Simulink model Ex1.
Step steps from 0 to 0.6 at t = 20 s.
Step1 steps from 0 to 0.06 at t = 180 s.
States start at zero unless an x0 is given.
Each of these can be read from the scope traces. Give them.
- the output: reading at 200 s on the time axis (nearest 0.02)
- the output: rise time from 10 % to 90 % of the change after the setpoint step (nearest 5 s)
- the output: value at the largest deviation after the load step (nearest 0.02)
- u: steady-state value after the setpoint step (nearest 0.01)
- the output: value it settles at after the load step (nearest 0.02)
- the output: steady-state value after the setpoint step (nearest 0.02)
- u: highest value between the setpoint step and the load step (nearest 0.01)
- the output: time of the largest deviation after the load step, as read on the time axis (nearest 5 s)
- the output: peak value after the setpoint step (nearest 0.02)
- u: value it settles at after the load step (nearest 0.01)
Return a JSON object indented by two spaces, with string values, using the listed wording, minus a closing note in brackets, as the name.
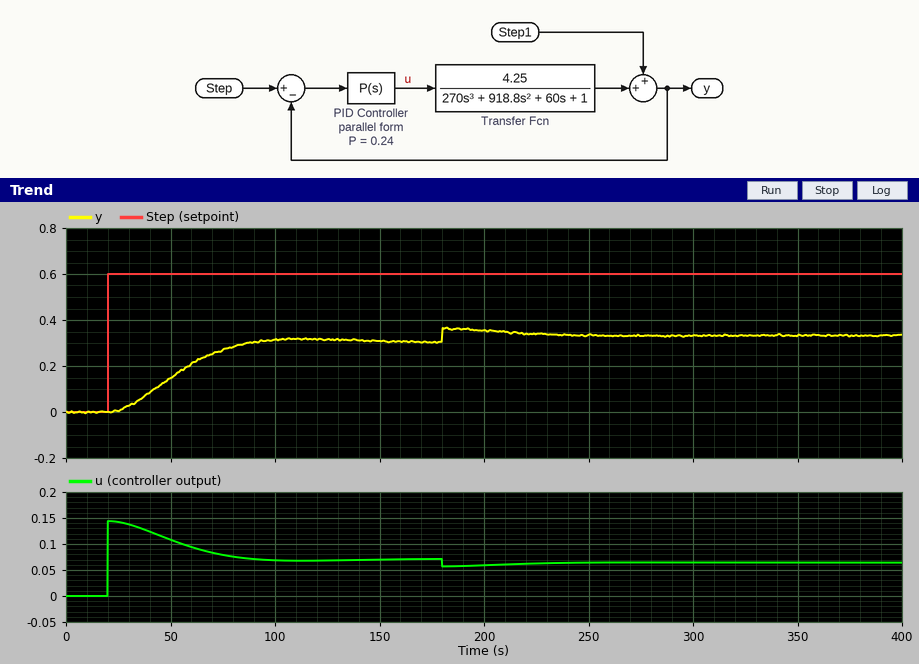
{
  "the output: reading at 200 s on the time axis": "0.36",
  "the output: rise time from 10 % to 90 % of the change after the setpoint step": "45 s",
  "the output: value at the largest deviation after the load step": "0.36",
  "u: steady-state value after the setpoint step": "0.07",
  "the output: value it settles at after the load step": "0.34",
  "the output: steady-state value after the setpoint step": "0.30",
  "u: highest value between the setpoint step and the load step": "0.14",
  "the output: time of the largest deviation after the load step, as read on the time axis": "180 s",
  "the output: peak value after the setpoint step": "0.32",
  "u: value it settles at after the load step": "0.06"
}
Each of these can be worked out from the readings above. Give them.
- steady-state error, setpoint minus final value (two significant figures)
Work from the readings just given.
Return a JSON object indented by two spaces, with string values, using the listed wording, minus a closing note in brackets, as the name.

{
  "steady-state error, setpoint minus final value": "0.30"
}
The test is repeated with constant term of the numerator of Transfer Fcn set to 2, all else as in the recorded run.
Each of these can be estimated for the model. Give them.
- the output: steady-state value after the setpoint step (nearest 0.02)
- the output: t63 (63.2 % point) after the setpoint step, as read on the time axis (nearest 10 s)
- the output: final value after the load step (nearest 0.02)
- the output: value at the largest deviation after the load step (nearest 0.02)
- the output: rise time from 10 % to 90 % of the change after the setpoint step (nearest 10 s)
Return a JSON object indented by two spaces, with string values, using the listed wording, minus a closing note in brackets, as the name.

{
  "the output: steady-state value after the setpoint step": "0.20",
  "the output: t63 (63.2 % point) after the setpoint step, as read on the time axis": "70 s",
  "the output: final value after the load step": "0.24",
  "the output: value at the largest deviation after the load step": "0.26",
  "the output: rise time from 10 % to 90 % of the change after the setpoint step": "60 s"
}
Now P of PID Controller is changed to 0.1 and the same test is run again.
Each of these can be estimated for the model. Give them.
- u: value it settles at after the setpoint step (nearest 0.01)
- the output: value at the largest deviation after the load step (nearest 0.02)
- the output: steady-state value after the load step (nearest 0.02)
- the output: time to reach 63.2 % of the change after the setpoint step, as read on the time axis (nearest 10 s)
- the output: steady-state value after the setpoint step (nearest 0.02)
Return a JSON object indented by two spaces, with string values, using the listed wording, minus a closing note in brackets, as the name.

{
  "u: value it settles at after the setpoint step": "0.04",
  "the output: value at the largest deviation after the load step": "0.24",
  "the output: steady-state value after the load step": "0.22",
  "the output: time to reach 63.2 % of the change after the setpoint step, as read on the time axis": "70 s",
  "the output: steady-state value after the setpoint step": "0.18"
}
